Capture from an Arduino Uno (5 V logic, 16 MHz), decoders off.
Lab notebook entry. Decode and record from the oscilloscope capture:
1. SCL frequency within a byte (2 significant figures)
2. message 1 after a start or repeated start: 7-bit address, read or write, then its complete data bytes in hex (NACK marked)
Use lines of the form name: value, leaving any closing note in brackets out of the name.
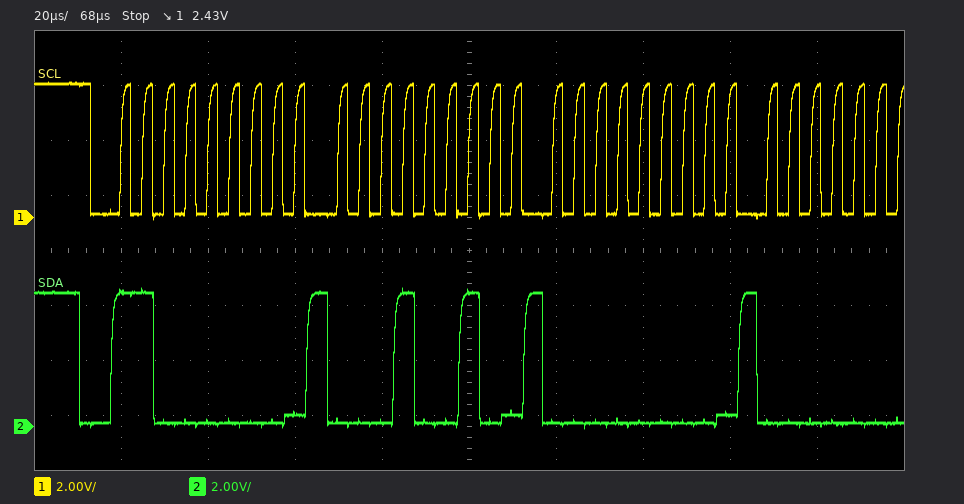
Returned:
SCL frequency within a byte: 200 kHz
message 1 after a start or repeated start: 7-bit address, read or write, then its complete data bytes in hex: 0x60 write: 12 00
